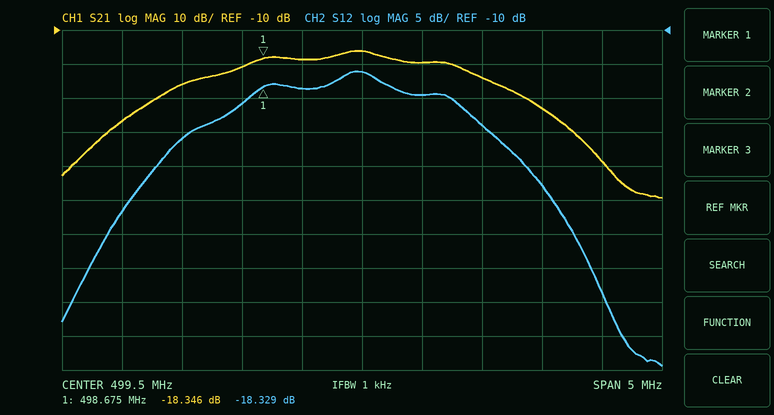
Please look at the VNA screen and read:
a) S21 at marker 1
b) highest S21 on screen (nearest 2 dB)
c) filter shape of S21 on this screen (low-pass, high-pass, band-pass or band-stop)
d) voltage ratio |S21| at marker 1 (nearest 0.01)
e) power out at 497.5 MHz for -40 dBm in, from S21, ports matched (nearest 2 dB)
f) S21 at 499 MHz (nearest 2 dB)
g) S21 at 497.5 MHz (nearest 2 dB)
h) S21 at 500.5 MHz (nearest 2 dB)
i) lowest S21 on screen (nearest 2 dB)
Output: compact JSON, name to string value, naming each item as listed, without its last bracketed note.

{"S21 at marker 1": "-18.346 dB", "highest S21 on screen": "-16 dB", "filter shape of S21 on this screen": "band-pass", "voltage ratio |S21| at marker 1": "0.12", "power out at 497.5 MHz for -40 dBm in, from S21, ports matched": "-76 dBm", "S21 at 499 MHz": "-18 dB", "S21 at 497.5 MHz": "-36 dB", "S21 at 500.5 MHz": "-24 dB", "lowest S21 on screen": "-60 dB"}
